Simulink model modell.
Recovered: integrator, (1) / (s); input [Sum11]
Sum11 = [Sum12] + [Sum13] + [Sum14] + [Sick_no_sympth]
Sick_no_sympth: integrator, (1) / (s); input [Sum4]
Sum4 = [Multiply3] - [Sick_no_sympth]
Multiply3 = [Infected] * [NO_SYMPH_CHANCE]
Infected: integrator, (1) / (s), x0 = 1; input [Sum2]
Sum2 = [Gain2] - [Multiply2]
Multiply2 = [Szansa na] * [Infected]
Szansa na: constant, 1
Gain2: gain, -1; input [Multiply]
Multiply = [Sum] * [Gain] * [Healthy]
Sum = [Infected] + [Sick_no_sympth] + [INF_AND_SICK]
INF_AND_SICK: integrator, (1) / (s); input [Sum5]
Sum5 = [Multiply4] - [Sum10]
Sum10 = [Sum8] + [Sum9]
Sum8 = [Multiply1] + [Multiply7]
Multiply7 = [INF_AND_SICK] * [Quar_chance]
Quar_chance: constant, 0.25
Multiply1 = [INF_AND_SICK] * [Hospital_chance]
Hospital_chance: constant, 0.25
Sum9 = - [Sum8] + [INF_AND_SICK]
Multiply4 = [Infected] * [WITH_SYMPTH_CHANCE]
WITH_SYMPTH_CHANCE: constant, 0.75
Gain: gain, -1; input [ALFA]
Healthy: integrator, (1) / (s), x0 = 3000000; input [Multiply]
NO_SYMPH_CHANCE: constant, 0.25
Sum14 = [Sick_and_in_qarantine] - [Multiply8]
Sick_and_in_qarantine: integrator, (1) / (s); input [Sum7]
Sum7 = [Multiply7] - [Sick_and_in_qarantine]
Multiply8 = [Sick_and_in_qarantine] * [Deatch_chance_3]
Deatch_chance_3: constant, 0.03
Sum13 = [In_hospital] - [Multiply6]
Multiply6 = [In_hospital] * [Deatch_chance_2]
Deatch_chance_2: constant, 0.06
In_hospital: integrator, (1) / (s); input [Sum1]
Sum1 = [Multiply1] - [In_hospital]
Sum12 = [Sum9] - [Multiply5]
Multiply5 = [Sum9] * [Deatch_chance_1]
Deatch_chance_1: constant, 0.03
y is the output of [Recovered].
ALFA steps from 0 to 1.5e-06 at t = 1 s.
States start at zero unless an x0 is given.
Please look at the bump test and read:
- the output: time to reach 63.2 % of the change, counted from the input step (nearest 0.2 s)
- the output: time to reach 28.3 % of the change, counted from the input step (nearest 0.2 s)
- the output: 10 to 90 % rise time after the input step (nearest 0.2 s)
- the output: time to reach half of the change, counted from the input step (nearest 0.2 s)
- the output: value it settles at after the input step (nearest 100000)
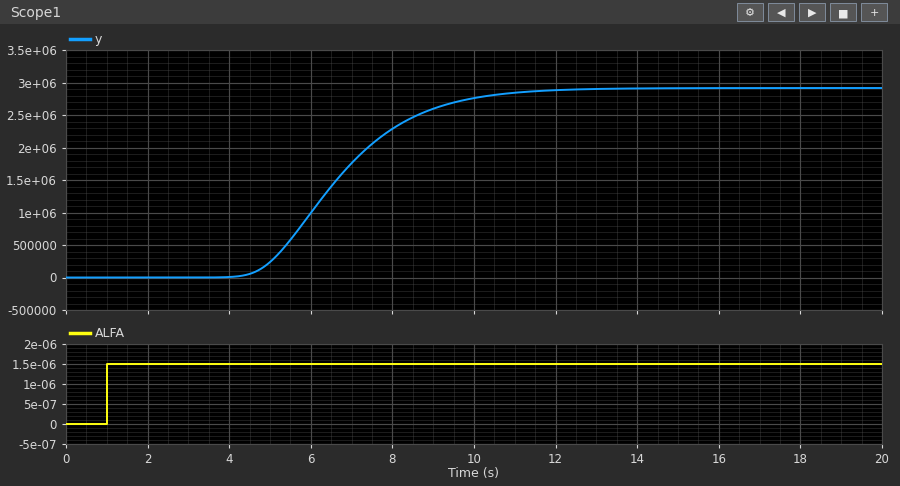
6.2 s
4.8 s
4.0 s
5.6 s
2900000
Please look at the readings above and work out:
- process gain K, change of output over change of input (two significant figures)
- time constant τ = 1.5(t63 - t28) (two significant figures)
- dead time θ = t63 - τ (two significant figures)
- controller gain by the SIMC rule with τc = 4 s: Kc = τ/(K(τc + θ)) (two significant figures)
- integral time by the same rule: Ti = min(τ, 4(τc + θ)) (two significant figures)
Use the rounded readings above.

1900000000000
2.1 s
4.1 s
0.00000000000014
2.1 s
